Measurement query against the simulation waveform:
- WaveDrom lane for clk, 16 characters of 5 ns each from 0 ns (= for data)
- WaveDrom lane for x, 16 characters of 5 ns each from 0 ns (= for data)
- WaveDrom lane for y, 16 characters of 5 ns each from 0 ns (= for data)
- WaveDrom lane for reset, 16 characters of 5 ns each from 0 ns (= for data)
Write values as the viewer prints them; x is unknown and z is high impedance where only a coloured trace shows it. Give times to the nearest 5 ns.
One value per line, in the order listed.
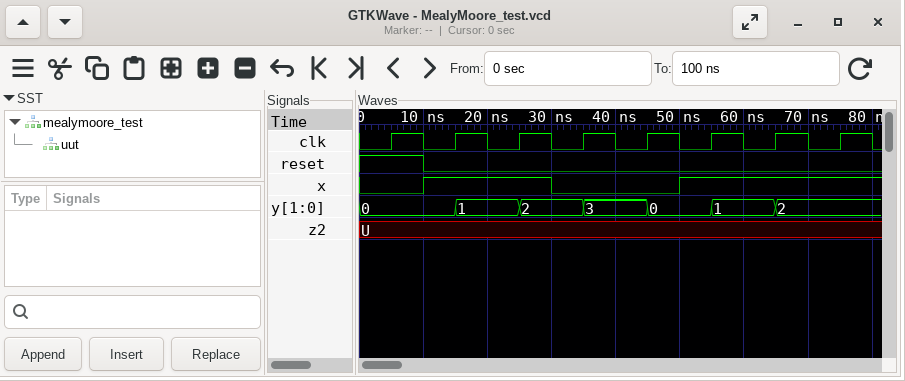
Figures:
{name: 'clk', wave: '0101010101010101'}
{name: 'x', wave: '0.1...0...1.....'}
{name: 'y', wave: '=..=.=.=.=.=.=..', data: '0 1 2 3 0 1 2'}
{name: 'reset', wave: '1.0.............'}
